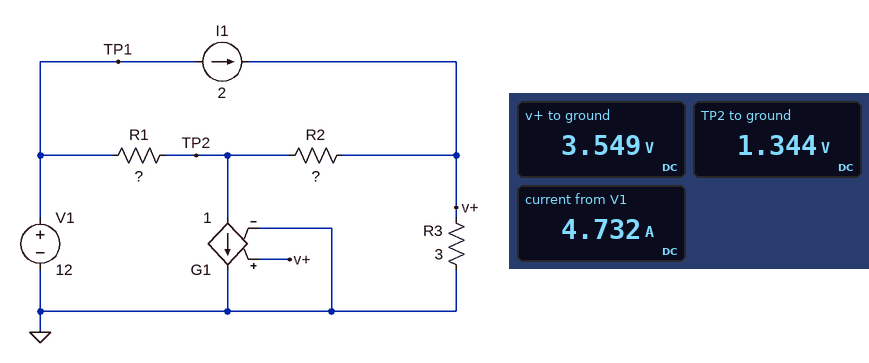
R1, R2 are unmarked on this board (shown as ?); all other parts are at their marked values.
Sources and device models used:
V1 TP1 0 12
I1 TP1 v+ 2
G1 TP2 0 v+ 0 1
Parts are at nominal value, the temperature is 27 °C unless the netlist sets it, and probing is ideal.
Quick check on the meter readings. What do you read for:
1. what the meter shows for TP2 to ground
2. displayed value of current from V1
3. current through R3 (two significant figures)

1.344 V
4.732 A
1.2 A
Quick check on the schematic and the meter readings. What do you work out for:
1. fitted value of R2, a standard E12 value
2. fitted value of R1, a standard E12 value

2.7 Ω
3.9 Ω
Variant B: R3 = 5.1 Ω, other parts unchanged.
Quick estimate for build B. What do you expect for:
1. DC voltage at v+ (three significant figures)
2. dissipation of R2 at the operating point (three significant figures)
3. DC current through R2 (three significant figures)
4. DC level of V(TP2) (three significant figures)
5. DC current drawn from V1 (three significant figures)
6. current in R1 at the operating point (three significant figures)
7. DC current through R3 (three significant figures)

4.07 V
3.90 W
1.20 A
822 mV
4.87 A
2.87 A
798 mA
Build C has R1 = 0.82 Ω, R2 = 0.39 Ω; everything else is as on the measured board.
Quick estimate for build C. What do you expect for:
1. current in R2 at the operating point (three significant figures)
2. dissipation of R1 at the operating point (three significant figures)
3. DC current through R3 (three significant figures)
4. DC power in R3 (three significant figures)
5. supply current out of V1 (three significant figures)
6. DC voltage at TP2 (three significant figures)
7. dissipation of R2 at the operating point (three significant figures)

162 mA
36.2 W
2.16 A
14.0 W
8.65 A
6.55 V
10.2 mW
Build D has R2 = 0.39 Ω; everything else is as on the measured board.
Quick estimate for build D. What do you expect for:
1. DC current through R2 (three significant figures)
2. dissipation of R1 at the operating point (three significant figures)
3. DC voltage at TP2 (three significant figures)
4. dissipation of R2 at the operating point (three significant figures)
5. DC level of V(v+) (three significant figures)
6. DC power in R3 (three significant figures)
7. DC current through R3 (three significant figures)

916 mA
21.3 W
2.89 V
327 mW
3.25 V
3.52 W
1.08 A
